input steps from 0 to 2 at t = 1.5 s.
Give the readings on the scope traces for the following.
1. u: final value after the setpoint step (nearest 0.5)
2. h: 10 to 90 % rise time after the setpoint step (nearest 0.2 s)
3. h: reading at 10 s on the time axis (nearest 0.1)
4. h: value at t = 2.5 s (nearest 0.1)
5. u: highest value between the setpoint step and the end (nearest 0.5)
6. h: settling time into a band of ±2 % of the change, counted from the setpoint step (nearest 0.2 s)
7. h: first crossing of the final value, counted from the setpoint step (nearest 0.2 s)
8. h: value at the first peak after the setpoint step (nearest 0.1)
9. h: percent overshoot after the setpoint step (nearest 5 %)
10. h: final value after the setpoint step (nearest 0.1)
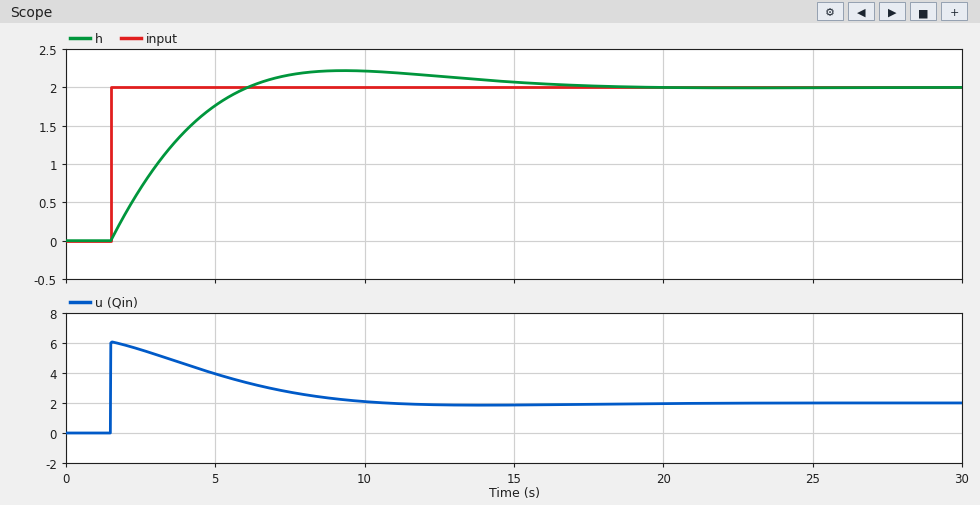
2.0
3.4 s
2.2
0.7
6.0
14.8 s
4.6 s
2.2
10 %
2.0
